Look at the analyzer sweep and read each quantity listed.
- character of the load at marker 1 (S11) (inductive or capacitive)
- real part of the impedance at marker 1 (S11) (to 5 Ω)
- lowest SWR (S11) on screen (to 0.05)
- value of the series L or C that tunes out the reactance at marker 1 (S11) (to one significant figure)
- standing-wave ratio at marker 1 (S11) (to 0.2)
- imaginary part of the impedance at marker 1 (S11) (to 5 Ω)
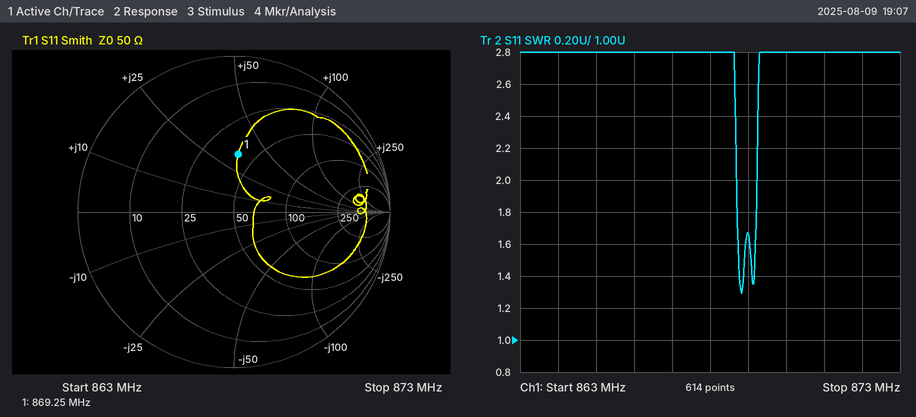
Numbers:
inductive
40 Ω
1.30
5 pF
2.2
+35 Ω
